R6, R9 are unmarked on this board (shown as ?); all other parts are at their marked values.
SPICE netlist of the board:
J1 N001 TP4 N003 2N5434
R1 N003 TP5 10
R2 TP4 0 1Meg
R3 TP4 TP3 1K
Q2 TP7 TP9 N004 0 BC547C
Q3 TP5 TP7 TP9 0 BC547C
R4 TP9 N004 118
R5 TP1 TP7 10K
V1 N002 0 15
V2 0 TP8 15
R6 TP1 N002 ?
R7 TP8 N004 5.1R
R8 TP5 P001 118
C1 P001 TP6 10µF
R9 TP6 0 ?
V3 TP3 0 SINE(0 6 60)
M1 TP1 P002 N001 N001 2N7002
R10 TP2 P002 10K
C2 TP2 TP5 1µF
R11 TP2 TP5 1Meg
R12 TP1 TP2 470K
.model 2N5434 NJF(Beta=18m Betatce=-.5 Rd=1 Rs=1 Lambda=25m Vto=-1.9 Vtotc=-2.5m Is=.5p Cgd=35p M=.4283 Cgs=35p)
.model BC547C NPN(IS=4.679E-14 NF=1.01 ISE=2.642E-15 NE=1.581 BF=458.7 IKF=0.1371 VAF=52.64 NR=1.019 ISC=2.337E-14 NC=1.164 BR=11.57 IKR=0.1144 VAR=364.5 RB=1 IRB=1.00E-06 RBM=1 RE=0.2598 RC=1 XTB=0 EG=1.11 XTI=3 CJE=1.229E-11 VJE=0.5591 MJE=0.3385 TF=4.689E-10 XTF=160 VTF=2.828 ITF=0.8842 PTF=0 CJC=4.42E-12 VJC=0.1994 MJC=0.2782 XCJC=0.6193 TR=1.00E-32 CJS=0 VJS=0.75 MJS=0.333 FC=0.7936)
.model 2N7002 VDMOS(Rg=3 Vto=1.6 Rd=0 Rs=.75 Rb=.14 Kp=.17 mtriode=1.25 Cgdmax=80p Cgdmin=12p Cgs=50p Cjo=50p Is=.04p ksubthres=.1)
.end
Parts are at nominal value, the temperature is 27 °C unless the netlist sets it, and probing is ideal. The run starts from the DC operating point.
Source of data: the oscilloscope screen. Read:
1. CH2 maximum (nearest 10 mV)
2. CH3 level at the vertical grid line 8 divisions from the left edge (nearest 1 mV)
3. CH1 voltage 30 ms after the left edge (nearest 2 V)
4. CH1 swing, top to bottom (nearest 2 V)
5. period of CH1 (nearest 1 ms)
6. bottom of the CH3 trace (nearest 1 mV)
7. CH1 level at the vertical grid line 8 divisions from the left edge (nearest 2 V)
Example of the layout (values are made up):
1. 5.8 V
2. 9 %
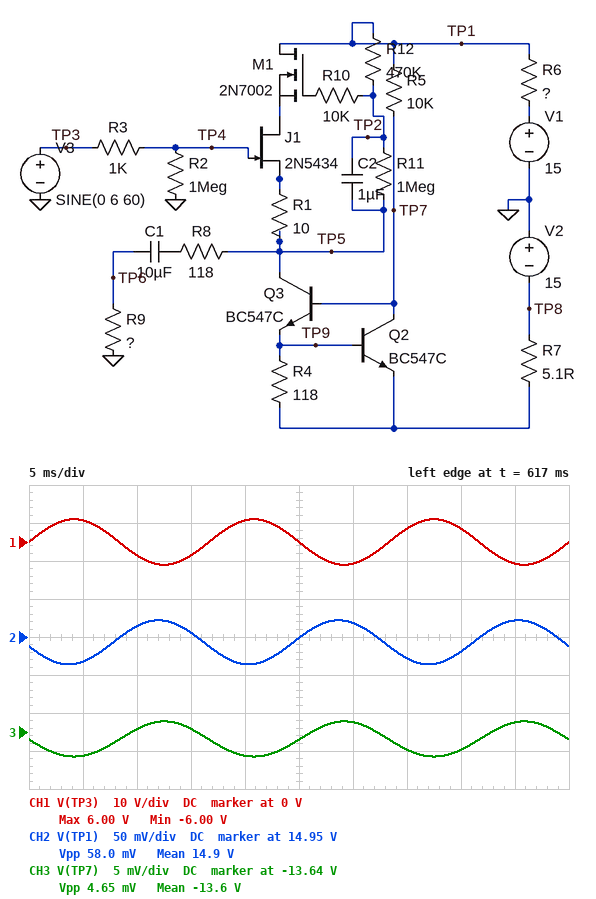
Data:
1. 14.97 V
2. -13.647 V
3. -6 V
4. 12 V
5. 17 ms
6. -13.648 V
7. 4 V
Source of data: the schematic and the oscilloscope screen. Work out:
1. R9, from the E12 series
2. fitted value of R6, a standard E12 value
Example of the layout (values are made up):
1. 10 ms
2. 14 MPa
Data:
1. 1.2 kΩ
2. 6.8 Ω
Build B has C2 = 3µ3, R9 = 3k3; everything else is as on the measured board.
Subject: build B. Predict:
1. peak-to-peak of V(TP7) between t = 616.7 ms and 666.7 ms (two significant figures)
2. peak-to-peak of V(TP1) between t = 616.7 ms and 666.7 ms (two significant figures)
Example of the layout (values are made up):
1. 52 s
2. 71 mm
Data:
1. 4.7 mV
2. 23 mV
